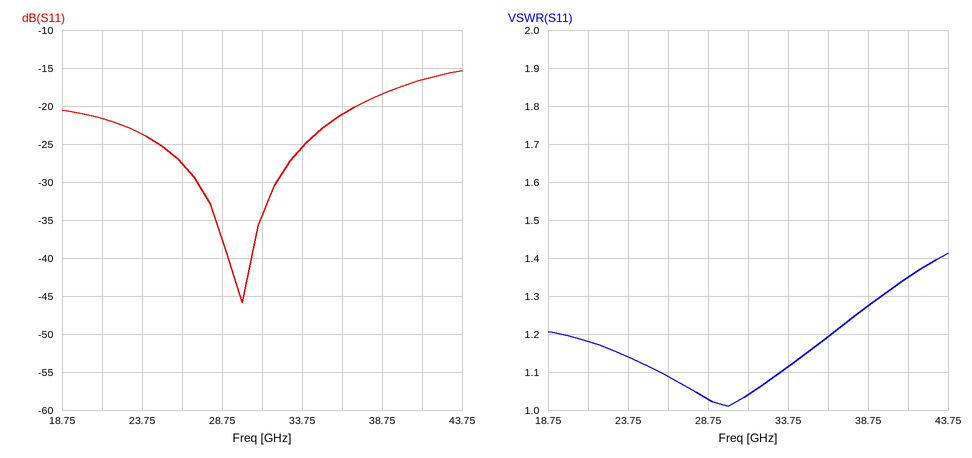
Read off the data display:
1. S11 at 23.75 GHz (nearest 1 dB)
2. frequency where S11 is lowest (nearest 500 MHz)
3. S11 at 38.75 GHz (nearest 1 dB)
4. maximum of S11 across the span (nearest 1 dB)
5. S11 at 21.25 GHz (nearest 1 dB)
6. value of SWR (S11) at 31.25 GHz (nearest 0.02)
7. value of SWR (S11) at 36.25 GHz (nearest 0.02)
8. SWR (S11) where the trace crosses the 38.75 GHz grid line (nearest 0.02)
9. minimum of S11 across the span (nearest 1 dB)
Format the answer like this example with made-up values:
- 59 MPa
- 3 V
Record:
- -24 dB
- 30.0 GHz
- -18 dB
- -15 dB
- -22 dB
- 1.04
- 1.20
- 1.28
- -46 dB
